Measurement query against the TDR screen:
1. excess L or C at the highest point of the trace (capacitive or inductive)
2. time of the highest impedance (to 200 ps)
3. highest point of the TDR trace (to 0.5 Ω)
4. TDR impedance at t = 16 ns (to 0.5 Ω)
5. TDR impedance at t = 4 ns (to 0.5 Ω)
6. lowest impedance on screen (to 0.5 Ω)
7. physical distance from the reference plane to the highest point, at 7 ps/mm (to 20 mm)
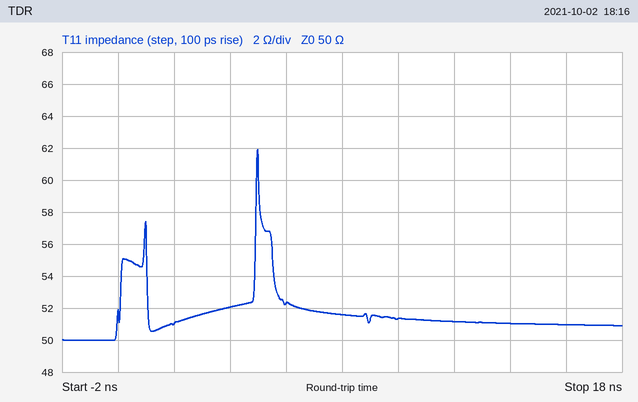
inductive
5.0 ns
62.0 Ω
51.0 Ω
52.0 Ω
50.0 Ω
360 mm
